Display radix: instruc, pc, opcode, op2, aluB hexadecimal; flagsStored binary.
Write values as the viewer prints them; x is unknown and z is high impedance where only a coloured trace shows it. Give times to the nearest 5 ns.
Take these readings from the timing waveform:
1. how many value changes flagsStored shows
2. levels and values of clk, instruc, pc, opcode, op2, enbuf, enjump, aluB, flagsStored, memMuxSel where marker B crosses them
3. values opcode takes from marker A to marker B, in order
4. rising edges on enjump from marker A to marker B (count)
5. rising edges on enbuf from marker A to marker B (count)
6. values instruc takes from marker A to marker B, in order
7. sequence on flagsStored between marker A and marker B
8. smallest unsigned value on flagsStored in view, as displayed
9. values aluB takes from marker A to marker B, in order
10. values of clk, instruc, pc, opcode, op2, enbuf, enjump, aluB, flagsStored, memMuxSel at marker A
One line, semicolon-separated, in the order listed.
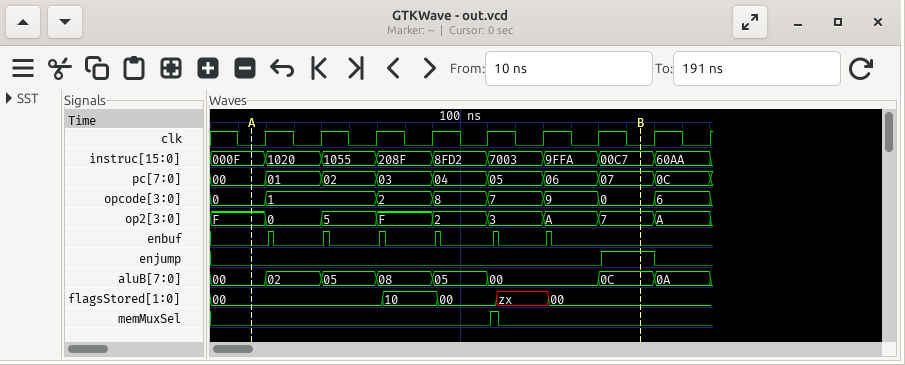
4; clk=0, instruc=00C7, pc=07, opcode=0, op2=7, enbuf=0, enjump=1, aluB=0C, flagsStored=00, memMuxSel=0; 0, 1, 2, 8, 7, 9, 0; 1; 6; 000F, 1020, 1055, 208F, 8FD2, 7003, 9FFA, 00C7; 00, 10, 00, zx, 00; 00; 00, 02, 05, 08, 05, 00, 0C; clk=0, instruc=000F, pc=00, opcode=0, op2=F, enbuf=0, enjump=0, aluB=00, flagsStored=00, memMuxSel=0
